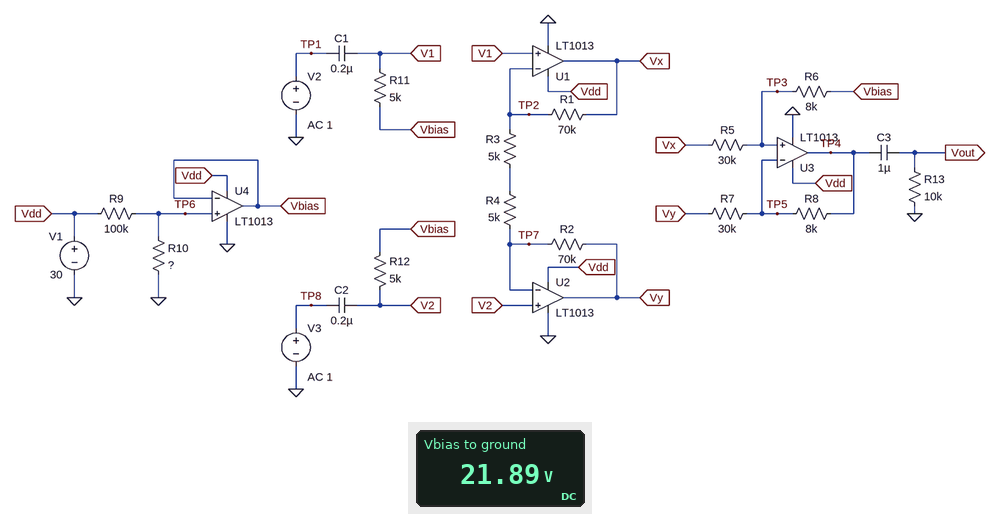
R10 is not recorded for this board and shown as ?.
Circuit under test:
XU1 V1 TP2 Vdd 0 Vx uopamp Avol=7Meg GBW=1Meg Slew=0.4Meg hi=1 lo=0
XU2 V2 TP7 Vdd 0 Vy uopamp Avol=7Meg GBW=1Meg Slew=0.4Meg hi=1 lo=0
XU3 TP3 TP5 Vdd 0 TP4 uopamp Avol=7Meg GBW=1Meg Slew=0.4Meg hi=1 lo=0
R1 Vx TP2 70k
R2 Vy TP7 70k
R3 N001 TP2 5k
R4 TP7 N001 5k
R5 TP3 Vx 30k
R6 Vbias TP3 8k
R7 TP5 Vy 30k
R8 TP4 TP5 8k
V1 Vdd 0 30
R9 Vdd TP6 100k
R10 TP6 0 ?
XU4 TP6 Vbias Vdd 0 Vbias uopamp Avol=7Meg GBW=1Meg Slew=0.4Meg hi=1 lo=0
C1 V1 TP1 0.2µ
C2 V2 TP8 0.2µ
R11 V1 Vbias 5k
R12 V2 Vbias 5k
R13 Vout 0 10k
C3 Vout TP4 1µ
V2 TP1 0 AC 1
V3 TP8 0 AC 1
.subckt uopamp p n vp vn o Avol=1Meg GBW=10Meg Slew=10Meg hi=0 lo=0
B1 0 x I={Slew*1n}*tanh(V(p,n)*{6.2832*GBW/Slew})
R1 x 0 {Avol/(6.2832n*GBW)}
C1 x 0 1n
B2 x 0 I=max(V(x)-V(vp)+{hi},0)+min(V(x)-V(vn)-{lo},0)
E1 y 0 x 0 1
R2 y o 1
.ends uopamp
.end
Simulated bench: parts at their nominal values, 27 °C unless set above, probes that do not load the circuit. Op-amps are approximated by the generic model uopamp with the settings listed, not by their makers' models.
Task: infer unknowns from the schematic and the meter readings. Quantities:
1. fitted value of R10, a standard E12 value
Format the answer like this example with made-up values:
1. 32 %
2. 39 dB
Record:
1. 270 kΩ
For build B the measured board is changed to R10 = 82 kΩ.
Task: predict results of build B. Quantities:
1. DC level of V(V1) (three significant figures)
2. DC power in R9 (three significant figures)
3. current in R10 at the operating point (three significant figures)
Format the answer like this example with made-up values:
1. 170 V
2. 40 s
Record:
1. 13.5 V
2. 2.72 mW
3. 165 µA
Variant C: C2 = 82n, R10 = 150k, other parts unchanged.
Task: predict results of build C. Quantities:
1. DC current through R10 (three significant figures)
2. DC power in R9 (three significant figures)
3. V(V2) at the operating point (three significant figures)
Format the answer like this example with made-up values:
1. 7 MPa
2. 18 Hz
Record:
1. 120 µA
2. 1.44 mW
3. 18.0 V
